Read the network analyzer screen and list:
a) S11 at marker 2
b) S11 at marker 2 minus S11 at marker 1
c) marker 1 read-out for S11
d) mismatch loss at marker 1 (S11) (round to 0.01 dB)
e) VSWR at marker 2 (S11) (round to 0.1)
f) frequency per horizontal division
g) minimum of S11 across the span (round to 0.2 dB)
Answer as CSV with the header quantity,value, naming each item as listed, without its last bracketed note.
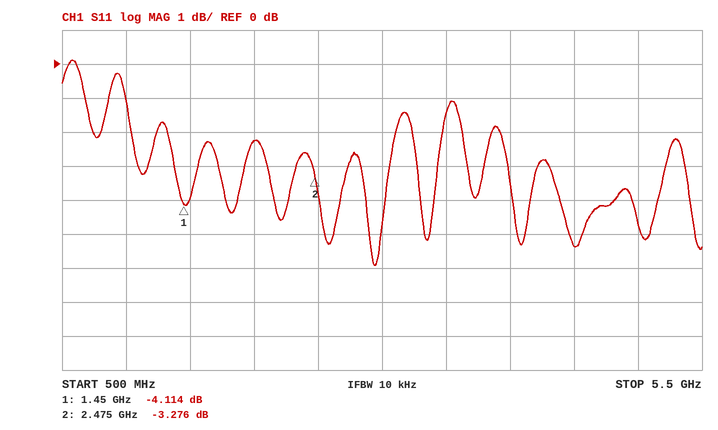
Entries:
quantity,value
S11 at marker 2,-3.276 dB
S11 at marker 2 minus S11 at marker 1,0.838 dB
marker 1 read-out for S11,-4.114 dB
mismatch loss at marker 1 (S11),2.13 dB
VSWR at marker 2 (S11),5.4
frequency per horizontal division,500 MHz
minimum of S11 across the span,-6.0 dB
